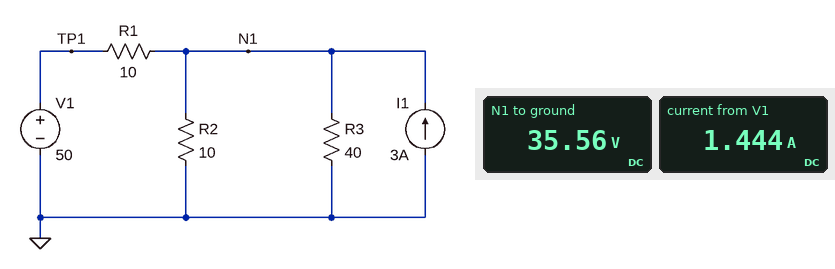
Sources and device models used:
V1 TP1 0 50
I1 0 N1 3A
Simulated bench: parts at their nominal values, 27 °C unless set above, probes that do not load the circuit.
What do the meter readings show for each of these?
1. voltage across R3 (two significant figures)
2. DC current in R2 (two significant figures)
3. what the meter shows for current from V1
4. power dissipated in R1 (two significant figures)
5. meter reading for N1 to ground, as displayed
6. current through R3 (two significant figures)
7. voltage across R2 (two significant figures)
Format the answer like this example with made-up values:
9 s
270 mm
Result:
36 V
3.6 A
1.444 A
21 W
35.56 V
890 mA
36 V
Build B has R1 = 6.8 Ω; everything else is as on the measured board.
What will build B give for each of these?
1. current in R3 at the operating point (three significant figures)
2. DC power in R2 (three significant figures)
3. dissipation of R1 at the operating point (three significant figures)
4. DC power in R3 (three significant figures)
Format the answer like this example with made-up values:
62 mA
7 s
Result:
951 mA
145 W
21.0 W
36.2 W
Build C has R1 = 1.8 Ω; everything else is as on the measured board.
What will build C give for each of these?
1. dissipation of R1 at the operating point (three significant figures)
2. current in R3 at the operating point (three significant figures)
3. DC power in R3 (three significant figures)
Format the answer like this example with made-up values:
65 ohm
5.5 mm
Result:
12.7 W
1.13 A
51.1 W
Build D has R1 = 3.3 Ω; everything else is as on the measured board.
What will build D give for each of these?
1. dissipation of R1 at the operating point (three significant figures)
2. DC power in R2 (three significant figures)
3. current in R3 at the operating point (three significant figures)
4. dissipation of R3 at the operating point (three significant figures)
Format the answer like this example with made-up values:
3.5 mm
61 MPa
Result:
17.5 W
180 W
1.06 A
45.0 W
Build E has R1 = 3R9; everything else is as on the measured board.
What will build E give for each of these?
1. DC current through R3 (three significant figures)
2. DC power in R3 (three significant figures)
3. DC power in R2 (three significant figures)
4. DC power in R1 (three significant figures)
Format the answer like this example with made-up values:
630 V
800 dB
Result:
1.04 A
43.0 W
172 W
18.6 W
